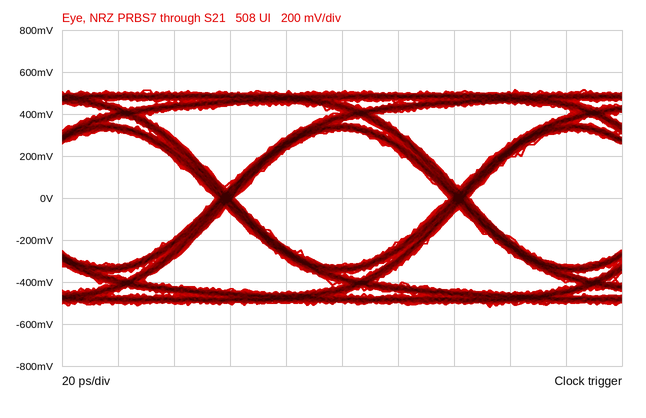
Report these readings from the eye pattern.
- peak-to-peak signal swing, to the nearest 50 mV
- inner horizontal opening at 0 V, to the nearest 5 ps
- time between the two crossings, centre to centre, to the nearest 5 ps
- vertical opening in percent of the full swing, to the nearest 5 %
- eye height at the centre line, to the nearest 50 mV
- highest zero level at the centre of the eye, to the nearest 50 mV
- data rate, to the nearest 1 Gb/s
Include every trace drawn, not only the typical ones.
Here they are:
1.05 V
75 ps
85 ps
60 %
650 mV
-300 mV
12 Gb/s
